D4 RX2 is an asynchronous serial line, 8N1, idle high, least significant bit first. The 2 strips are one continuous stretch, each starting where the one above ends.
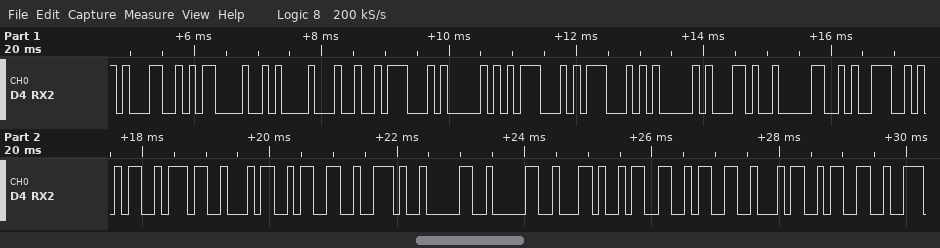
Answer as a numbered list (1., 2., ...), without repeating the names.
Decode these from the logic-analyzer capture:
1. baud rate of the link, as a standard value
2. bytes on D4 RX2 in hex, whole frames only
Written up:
1. 9600 baud
2. 31 0D 0A 24 47 50 47 47 41 2C 30 39 35 37 34 33 2E 30 30 2C 33 33 34 33
